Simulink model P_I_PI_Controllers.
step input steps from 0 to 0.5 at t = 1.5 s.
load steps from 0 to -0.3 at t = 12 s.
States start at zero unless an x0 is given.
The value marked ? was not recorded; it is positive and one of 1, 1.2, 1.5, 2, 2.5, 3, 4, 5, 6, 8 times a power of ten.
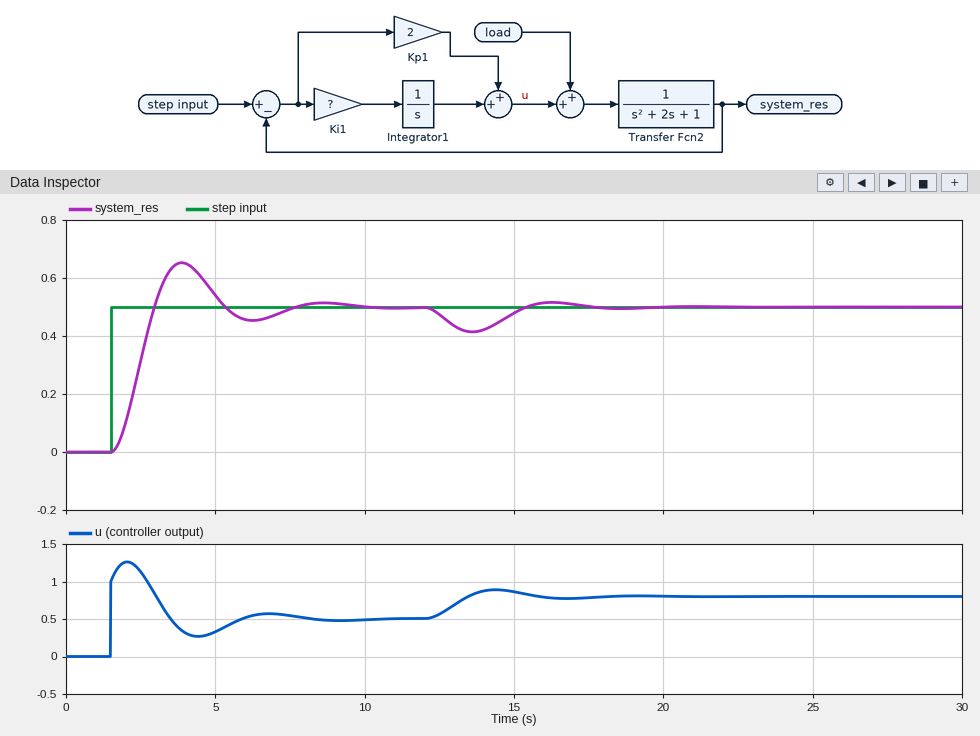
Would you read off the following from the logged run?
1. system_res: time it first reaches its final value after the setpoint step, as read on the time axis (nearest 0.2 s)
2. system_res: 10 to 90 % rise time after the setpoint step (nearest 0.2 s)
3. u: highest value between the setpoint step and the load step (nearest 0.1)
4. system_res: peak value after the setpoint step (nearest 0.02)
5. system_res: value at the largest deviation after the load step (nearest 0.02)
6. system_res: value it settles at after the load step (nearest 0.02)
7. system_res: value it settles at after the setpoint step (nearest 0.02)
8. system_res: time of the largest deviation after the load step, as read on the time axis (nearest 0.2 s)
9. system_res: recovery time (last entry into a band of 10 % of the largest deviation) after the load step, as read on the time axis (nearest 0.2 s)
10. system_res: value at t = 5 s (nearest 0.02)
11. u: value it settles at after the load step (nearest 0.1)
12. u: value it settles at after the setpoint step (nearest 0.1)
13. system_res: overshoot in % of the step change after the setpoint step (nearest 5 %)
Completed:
3.0 s
1.0 s
1.3
0.66
0.42
0.50
0.50
13.6 s
17.0 s
0.54
0.8
0.5
30 %
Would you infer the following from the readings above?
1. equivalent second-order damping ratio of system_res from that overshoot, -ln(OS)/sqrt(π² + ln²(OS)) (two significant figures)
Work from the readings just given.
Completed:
0.36
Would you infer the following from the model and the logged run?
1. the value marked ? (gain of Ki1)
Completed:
2
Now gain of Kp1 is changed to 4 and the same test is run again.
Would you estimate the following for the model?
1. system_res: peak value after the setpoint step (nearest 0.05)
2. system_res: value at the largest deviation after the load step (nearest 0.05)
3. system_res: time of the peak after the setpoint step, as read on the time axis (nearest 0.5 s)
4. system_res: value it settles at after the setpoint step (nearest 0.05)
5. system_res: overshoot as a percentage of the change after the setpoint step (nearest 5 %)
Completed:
0.60
0.45
3.0 s
0.50
25 %
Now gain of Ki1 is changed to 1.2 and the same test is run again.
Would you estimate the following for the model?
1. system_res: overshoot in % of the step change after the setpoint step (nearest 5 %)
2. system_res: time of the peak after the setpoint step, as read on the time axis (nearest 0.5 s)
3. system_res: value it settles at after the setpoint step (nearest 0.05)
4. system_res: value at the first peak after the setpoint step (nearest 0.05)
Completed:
10 %
4.0 s
0.50
0.55
